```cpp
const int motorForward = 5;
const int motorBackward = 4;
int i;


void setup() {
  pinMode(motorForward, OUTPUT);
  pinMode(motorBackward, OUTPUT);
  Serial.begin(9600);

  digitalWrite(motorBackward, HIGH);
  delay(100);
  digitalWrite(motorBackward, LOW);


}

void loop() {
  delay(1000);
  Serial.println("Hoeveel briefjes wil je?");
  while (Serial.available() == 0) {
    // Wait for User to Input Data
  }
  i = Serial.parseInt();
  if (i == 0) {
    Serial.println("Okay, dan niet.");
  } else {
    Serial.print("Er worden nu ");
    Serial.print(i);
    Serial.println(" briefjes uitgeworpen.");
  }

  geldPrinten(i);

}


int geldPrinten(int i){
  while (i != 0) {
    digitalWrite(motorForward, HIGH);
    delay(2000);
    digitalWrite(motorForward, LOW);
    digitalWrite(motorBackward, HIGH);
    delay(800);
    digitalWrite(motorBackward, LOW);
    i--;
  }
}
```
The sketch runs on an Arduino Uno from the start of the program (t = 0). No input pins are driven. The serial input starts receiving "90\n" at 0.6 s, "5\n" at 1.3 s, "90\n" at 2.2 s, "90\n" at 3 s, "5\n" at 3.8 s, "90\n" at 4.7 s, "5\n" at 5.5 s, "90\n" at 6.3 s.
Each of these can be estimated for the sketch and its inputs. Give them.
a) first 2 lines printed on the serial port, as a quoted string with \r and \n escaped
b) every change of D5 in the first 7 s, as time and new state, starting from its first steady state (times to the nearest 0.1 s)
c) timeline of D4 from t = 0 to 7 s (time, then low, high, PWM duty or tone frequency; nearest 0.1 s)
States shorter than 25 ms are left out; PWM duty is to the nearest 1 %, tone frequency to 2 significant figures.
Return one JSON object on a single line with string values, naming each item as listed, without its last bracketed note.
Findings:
{"first 2 lines printed on the serial port, as a quoted string with \\r and \\n escaped": "\"Hoeveel briefjes wil je?\\r\\nEr worden nu 90 briefjes uitgeworpen.\\r\\n\"", "every change of D5 in the first 7 s, as time and new state, starting from its first steady state": "0 s low; 1.1 s high; 3.1 s low; 3.9 s high; 5.9 s low; 6.7 s high", "timeline of D4 from t = 0 to 7 s": "0 s high; 0.1 s low; 3.1 s high; 3.9 s low; 5.9 s high; 6.7 s low"}
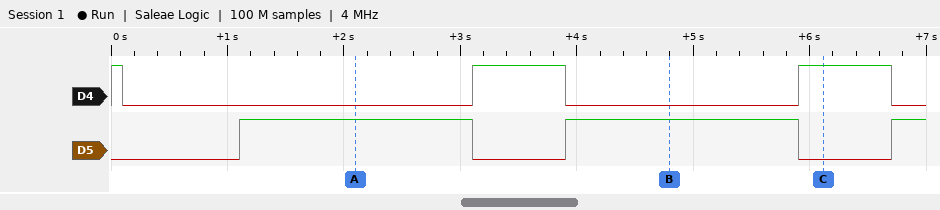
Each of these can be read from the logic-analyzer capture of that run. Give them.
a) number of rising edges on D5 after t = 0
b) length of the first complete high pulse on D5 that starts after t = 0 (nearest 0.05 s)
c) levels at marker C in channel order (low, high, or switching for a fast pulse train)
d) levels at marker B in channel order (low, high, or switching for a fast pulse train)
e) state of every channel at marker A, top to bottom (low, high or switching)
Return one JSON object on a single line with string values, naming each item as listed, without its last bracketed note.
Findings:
{"number of rising edges on D5 after t = 0": "3", "length of the first complete high pulse on D5 that starts after t = 0": "2.00 s", "levels at marker C in channel order": "D4 high, D5 low", "levels at marker B in channel order": "D4 low, D5 high", "state of every channel at marker A, top to bottom": "D4 low, D5 high"}
